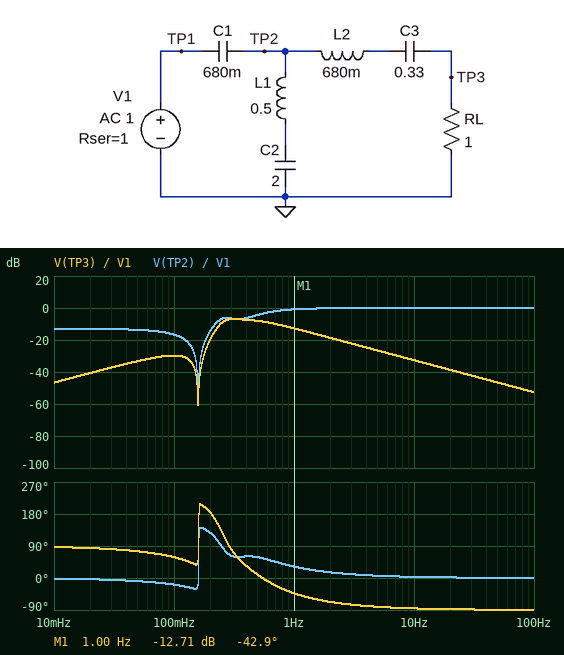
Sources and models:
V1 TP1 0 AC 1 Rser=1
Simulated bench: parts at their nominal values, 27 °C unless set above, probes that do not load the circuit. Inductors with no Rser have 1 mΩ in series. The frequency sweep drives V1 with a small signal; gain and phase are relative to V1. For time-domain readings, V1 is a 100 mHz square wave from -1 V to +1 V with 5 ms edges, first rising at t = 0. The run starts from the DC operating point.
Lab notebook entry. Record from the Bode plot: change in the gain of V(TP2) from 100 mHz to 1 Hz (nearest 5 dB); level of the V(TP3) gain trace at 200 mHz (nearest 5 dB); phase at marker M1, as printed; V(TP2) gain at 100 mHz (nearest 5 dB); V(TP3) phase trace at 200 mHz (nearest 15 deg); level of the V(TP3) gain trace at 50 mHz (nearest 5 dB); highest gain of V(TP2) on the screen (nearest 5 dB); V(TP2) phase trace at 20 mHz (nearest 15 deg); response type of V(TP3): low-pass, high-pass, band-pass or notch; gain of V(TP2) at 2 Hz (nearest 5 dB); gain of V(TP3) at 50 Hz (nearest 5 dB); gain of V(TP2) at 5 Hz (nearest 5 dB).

15 dB
-20 dB
-42.9 deg
-15 dB
180 deg
-35 dB
0 dB
0 deg
band-pass
0 dB
-45 dB
0 dB
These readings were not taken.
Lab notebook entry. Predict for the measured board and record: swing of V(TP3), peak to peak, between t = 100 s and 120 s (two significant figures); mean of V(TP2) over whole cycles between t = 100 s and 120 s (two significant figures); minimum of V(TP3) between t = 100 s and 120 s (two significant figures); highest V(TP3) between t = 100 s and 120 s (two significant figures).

880 mV
230 mV
-440 mV
440 mV
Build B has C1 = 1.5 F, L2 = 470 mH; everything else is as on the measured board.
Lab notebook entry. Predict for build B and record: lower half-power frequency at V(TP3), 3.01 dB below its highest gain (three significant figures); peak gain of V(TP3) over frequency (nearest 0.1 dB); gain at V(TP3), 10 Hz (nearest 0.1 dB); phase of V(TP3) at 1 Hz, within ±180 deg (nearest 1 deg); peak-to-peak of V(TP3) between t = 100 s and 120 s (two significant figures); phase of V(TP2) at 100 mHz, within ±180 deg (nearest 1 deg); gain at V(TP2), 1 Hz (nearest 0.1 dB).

253 mHz
-6.4 dB
-29.4 dB
-35 deg
1.0 V
-33 deg
-2.1 dB
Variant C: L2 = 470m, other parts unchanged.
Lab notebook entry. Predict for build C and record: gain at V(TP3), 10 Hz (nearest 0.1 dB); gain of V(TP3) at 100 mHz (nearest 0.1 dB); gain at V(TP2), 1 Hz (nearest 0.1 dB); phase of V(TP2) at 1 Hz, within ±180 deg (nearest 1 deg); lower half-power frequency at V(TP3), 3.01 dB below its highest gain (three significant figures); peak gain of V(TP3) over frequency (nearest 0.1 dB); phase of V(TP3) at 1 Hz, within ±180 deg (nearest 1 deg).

-29.4 dB
-29.9 dB
-1.7 dB
36 deg
256 mHz
-6.3 dB
-32 deg
